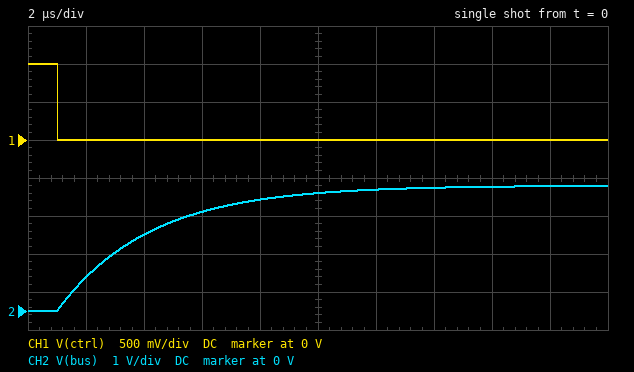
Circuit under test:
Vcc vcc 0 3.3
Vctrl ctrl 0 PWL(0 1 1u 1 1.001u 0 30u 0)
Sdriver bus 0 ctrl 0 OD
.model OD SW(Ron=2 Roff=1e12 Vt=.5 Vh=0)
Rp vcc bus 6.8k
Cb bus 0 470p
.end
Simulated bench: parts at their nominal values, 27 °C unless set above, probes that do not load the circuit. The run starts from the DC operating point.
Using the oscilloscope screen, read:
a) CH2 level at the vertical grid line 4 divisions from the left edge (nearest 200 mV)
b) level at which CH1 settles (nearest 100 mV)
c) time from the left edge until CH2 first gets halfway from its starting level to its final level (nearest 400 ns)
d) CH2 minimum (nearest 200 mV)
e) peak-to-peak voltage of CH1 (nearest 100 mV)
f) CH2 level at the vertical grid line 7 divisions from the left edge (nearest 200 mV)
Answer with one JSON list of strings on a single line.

["3.0 V", "0 V", "3.2 µs", "0 V", "1.0 V", "3.2 V"]
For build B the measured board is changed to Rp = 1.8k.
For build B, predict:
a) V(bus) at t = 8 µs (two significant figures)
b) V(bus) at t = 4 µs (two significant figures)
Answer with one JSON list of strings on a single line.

["3.3 V", "3.2 V"]
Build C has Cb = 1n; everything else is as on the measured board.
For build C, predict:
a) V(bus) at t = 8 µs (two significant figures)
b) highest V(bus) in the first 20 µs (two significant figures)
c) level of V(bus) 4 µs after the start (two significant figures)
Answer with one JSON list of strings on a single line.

["2.1 V", "3.1 V", "1.2 V"]
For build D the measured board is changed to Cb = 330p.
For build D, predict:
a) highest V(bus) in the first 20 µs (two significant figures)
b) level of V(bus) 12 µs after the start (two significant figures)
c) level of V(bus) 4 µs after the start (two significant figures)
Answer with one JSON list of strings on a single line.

["3.3 V", "3.3 V", "2.4 V"]
